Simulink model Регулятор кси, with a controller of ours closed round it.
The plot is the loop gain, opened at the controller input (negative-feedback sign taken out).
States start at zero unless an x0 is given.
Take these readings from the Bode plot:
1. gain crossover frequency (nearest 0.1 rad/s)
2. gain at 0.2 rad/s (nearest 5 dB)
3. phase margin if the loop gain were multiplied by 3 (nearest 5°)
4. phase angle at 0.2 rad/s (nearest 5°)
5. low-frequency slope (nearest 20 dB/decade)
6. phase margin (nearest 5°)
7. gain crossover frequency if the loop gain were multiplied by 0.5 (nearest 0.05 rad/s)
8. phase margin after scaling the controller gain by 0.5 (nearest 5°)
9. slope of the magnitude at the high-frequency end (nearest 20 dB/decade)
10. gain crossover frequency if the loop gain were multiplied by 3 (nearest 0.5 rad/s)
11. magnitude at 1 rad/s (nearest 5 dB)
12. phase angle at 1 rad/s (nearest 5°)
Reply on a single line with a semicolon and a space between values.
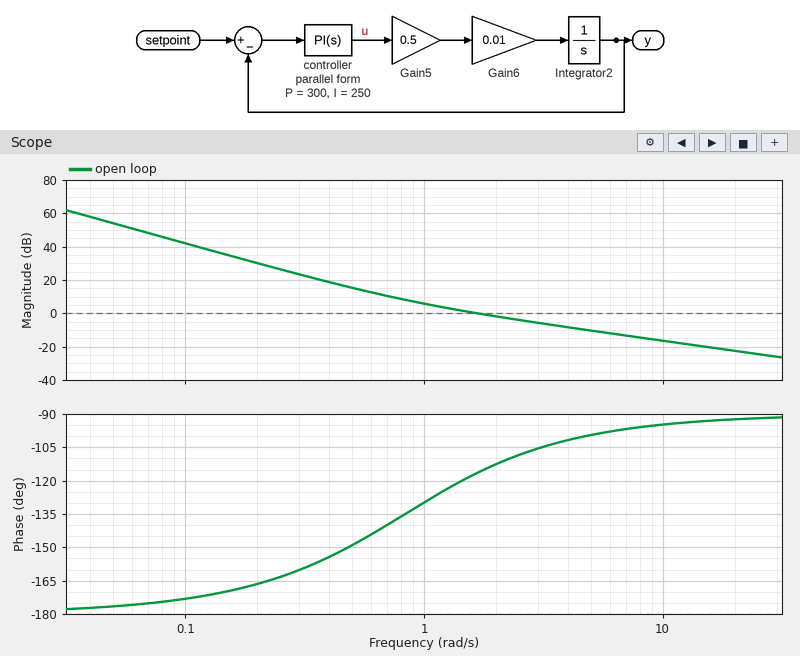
1.7 rad/s; 30 dB; 80°; -165°; -40 dB/decade; 65°; 1.00 rad/s; 50°; -20 dB/decade; 4.5 rad/s; 5 dB; -130°
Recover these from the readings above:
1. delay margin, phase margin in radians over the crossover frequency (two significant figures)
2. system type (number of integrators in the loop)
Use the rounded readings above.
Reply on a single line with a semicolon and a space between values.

0.67 s; 2
